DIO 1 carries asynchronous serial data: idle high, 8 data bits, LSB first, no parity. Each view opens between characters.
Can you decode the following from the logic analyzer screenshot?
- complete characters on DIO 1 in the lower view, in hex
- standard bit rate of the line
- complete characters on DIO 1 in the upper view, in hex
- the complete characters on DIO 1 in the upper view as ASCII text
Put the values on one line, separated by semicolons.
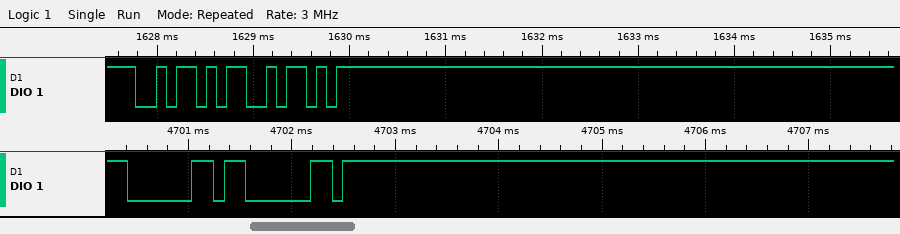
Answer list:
60, 60; 9600 baud; 5A, 5A; "ZZ"
